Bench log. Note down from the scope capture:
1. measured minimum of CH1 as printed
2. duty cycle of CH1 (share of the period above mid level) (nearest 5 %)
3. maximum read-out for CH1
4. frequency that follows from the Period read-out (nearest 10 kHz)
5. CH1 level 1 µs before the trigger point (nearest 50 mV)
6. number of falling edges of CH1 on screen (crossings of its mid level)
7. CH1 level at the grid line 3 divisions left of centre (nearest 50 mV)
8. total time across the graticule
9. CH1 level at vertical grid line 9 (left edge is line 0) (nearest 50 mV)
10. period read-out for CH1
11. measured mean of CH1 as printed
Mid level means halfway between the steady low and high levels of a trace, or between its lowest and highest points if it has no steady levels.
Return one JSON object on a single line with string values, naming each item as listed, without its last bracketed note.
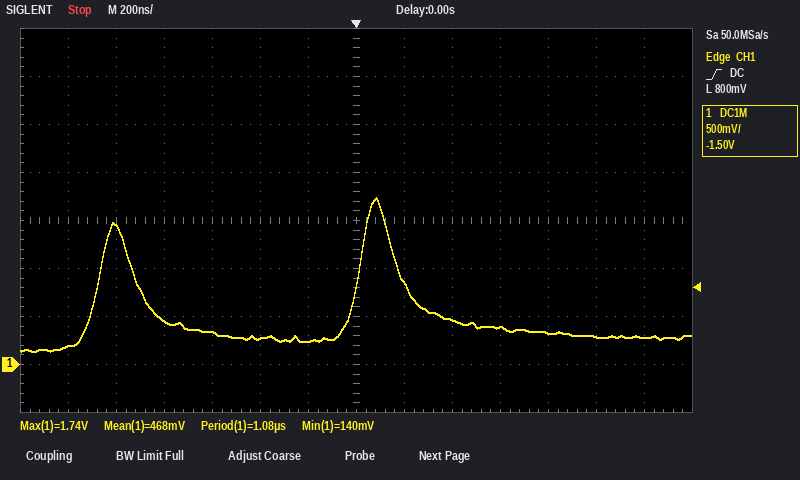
{"measured minimum of CH1 as printed": "140 mV", "duty cycle of CH1 (share of the period above mid level)": "15 %", "maximum read-out for CH1": "1.74 V", "frequency that follows from the Period read-out": "930 kHz", "CH1 level 1 µs before the trigger point": "1.45 V", "number of falling edges of CH1 on screen": "2", "CH1 level at the grid line 3 divisions left of centre": "350 mV", "total time across the graticule": "2.8 µs", "CH1 level at vertical grid line 9 (left edge is line 0)": "450 mV", "period read-out for CH1": "1.08 µs", "measured mean of CH1 as printed": "468 mV"}
